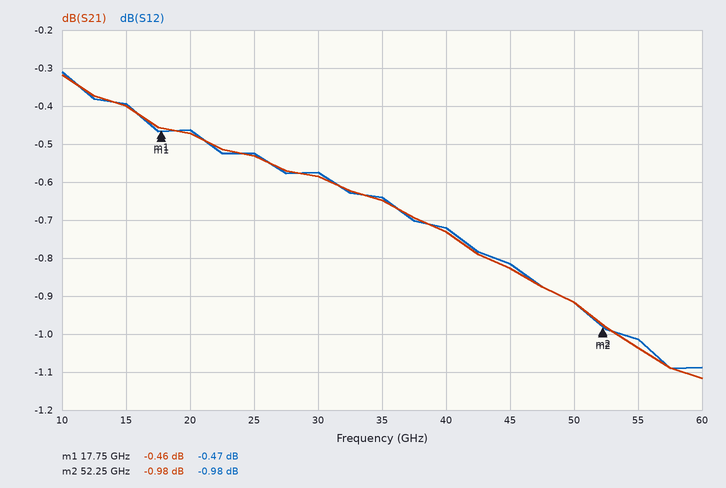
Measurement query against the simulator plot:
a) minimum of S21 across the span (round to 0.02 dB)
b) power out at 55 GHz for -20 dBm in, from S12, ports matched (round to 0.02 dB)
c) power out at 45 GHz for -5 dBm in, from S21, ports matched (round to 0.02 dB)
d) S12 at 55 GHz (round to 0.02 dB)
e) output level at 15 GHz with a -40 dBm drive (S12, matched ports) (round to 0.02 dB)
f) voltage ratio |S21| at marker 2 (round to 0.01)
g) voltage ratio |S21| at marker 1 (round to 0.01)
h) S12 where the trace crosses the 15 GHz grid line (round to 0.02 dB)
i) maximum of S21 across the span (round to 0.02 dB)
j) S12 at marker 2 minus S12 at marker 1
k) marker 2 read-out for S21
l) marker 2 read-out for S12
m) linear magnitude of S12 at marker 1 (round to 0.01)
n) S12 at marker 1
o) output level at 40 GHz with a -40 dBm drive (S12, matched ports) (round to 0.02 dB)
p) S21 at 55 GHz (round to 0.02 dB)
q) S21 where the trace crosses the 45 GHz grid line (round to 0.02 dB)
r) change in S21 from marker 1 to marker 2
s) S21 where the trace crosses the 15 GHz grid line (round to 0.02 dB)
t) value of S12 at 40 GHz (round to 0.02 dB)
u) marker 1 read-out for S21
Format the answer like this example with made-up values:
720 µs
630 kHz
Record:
-1.12 dB
-21.02 dBm
-5.82 dBm
-1.02 dB
-40.40 dBm
0.89
0.95
-0.40 dB
-0.32 dB
-0.51 dB
-0.98 dB
-0.98 dB
0.95
-0.47 dB
-40.72 dBm
-1.04 dB
-0.82 dB
-0.52 dB
-0.40 dB
-0.72 dB
-0.46 dB
